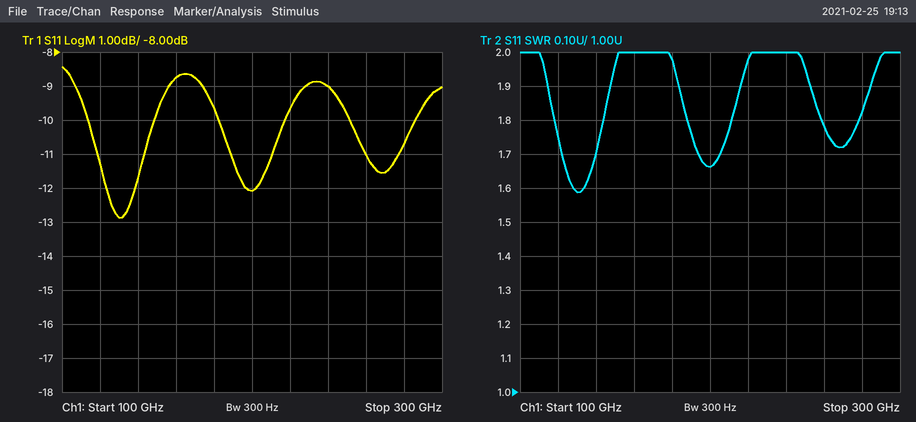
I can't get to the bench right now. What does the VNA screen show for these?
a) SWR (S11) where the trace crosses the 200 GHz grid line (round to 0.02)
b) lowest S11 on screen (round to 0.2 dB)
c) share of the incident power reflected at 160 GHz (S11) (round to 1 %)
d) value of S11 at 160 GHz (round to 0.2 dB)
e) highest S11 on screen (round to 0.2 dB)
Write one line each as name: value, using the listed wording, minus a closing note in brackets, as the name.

SWR (S11) where the trace crosses the 200 GHz grid line: 1.66
lowest S11 on screen: -12.8 dB
share of the incident power reflected at 160 GHz (S11): 13 %
value of S11 at 160 GHz: -8.8 dB
highest S11 on screen: -8.4 dB
